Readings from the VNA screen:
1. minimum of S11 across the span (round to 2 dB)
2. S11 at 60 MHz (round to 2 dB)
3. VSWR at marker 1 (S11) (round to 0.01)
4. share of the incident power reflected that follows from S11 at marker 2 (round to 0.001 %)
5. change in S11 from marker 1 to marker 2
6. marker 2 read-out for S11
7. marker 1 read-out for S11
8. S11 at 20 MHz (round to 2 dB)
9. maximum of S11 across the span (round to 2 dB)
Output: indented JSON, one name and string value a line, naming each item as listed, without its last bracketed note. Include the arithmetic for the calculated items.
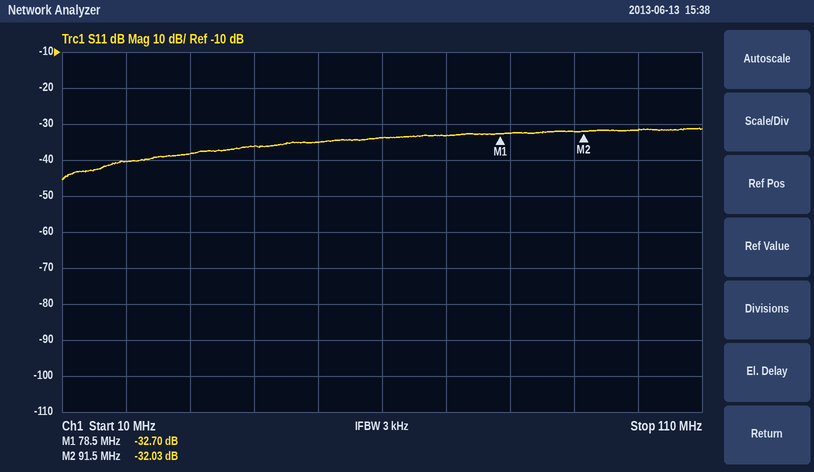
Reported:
{
  "minimum of S11 across the span": "-46 dB",
  "S11 at 60 MHz": "-34 dB",
  "VSWR at marker 1 (S11)": "(1 + 0.0232)/(1 − 0.0232) ≈ 1.05",
  "share of the incident power reflected that follows from S11 at marker 2": "10^(-32.03/10) ≈ 0.063 %",
  "change in S11 from marker 1 to marker 2": "-32.03 − (-32.7) = 0.67 dB",
  "marker 2 read-out for S11": "-32.03 dB",
  "marker 1 read-out for S11": "-32.70 dB",
  "S11 at 20 MHz": "-40 dB",
  "maximum of S11 across the span": "-32 dB"
}
